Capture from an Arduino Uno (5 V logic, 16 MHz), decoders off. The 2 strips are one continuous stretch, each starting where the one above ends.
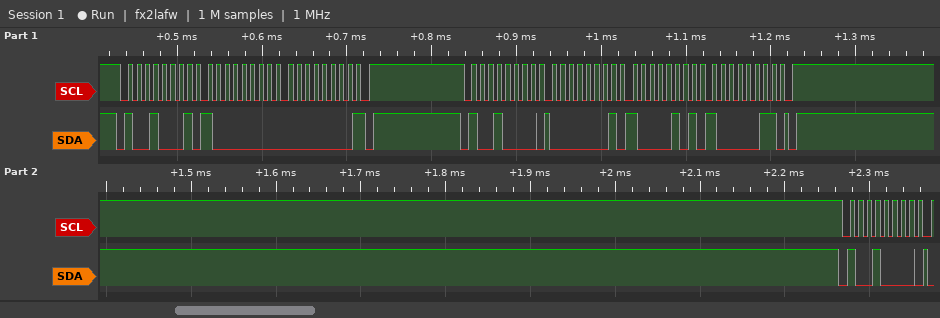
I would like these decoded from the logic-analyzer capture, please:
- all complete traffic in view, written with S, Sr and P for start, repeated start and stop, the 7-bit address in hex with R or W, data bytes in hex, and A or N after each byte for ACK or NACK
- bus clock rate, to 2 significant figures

S 48R A 80 A 00 N P S 48W A 01 A 85 A 83 A P S 48W A
100 kHz
